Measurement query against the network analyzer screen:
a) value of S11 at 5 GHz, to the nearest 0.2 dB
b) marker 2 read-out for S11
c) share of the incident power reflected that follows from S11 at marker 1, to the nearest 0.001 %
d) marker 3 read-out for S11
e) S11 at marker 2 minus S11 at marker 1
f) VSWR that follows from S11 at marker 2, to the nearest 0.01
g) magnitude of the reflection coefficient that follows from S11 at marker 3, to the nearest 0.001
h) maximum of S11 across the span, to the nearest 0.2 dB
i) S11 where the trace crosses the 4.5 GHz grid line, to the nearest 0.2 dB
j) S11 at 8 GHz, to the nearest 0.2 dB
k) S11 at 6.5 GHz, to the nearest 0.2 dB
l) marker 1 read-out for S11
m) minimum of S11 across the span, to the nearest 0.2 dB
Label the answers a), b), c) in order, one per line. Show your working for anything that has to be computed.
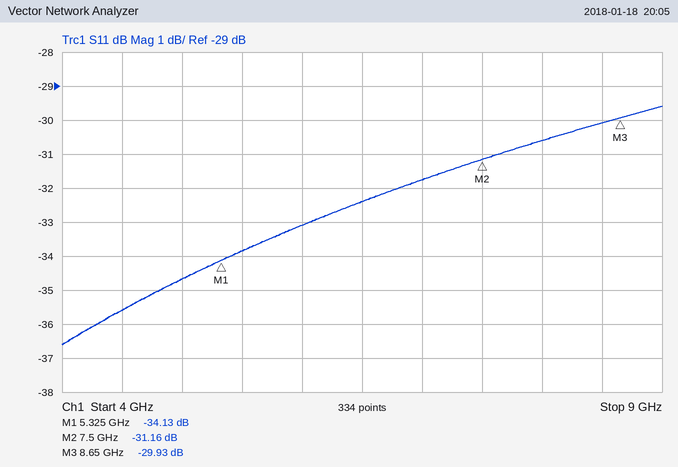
a) -34.6 dB
b) -31.16 dB
c) 10^(-34.13/10) ≈ 0.039 %
d) -29.93 dB
e) -31.16 − (-34.13) = 2.97 dB
f) (1 + 0.0277)/(1 − 0.0277) ≈ 1.06
g) 10^(-29.93/20) ≈ 0.032
h) -29.6 dB
i) -35.6 dB
j) -30.6 dB
k) -32.4 dB
l) -34.13 dB
m) -36.6 dB
